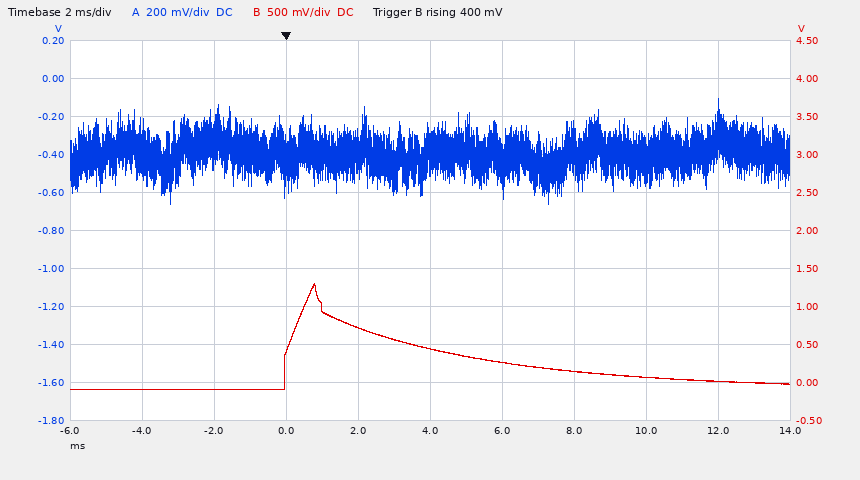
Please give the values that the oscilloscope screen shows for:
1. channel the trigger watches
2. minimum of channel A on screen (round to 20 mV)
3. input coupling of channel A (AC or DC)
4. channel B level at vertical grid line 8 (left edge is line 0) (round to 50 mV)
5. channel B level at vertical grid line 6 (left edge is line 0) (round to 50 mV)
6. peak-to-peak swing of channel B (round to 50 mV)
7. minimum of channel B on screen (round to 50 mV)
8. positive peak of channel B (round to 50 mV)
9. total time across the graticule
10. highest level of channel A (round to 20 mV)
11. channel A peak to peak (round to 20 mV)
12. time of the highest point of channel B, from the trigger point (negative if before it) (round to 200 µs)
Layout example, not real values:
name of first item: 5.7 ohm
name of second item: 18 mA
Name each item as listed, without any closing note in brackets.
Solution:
channel the trigger watches: channel B
minimum of channel A on screen: -660 mV
input coupling of channel A: DC
channel B level at vertical grid line 8 (left edge is line 0): 50 mV
channel B level at vertical grid line 6 (left edge is line 0): 250 mV
peak-to-peak swing of channel B: 1.40 V
minimum of channel B on screen: -100 mV
positive peak of channel B: 1.30 V
total time across the graticule: 20 ms
highest level of channel A: -100 mV
channel A peak to peak: 560 mV
time of the highest point of channel B, from the trigger point (negative if before it): +800 µs
